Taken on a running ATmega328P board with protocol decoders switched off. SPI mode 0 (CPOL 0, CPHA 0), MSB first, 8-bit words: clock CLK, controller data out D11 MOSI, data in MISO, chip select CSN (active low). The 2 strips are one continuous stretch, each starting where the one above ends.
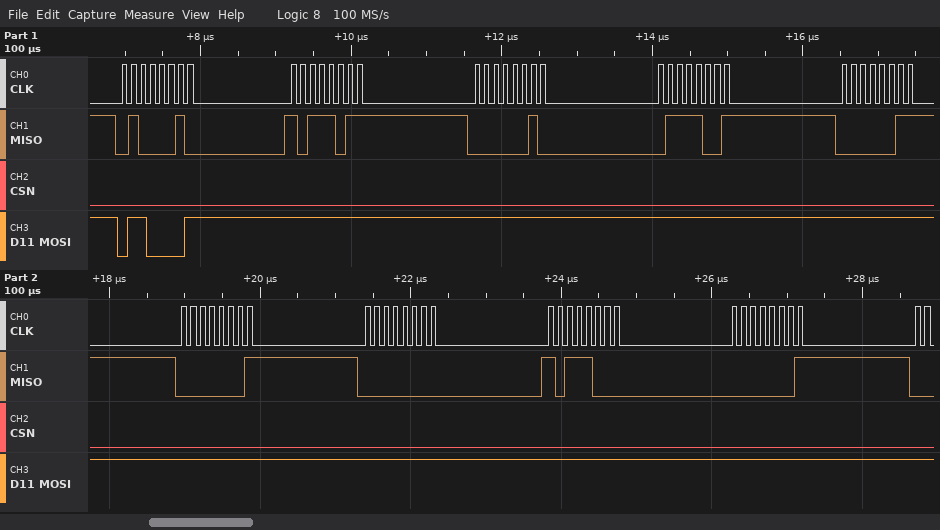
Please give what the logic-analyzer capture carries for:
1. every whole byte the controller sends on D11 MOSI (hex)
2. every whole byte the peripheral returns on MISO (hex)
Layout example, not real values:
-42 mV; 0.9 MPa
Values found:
61 FF FF FF FF FF FF FF FF; 42 BB 02 79 03 01 00 B8 01
